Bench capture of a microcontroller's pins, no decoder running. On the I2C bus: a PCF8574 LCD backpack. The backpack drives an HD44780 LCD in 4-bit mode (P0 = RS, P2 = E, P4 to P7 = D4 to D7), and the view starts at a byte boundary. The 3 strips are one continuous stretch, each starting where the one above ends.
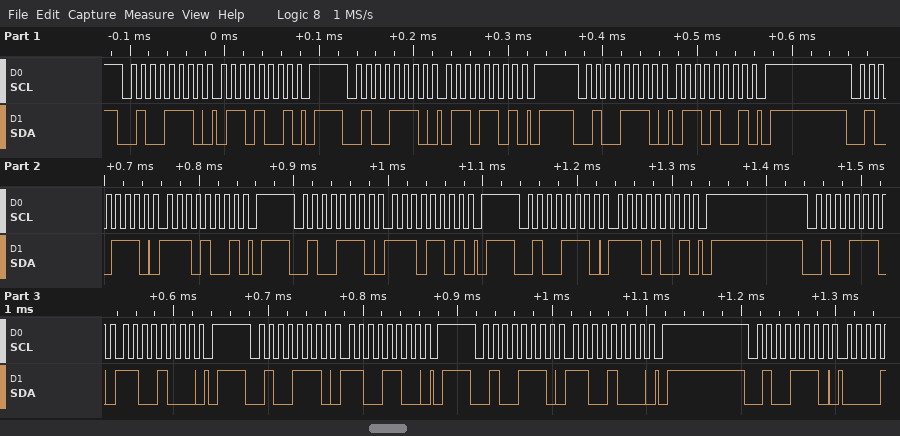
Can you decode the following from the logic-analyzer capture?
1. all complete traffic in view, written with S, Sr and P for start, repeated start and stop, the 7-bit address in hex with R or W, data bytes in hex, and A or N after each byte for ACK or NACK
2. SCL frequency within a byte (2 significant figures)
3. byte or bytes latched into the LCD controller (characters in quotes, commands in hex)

S 27W A 69 A P S 27W A 6D A P S 27W A 69 A P S 27W A E9 A P S 27W A ED A P S 27W A E9 A P S 27W A C8 A P S 27W A CC A P S 27W A C8 A P S 27W A
100 kHz
'n'
